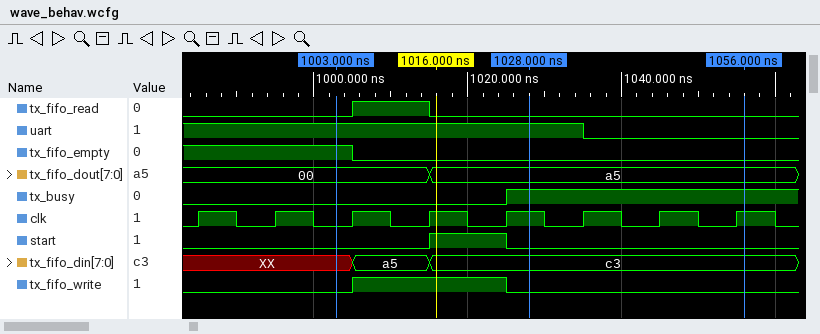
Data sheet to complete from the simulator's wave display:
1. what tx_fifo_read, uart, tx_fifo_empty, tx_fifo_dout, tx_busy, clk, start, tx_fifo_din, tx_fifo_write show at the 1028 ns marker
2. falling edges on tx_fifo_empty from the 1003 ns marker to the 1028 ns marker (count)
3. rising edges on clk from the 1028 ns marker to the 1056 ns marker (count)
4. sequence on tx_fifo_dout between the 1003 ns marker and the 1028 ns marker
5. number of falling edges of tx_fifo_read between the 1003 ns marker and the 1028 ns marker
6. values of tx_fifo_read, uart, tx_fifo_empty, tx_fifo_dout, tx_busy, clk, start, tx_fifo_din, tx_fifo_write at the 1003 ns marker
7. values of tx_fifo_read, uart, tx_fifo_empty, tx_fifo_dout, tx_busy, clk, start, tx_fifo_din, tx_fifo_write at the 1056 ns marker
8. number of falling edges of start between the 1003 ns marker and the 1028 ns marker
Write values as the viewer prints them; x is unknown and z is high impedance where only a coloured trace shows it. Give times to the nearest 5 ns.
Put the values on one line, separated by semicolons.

tx_fifo_read=0, uart=1, tx_fifo_empty=0, tx_fifo_dout=a5, tx_busy=1, clk=1, start=0, tx_fifo_din=c3, tx_fifo_write=0; 1; 3; 00, a5; 1; tx_fifo_read=0, uart=1, tx_fifo_empty=1, tx_fifo_dout=00, tx_busy=0, clk=0, start=0, tx_fifo_din=XX, tx_fifo_write=0; tx_fifo_read=0, uart=0, tx_fifo_empty=0, tx_fifo_dout=a5, tx_busy=1, clk=1, start=0, tx_fifo_din=c3, tx_fifo_write=0; 1
